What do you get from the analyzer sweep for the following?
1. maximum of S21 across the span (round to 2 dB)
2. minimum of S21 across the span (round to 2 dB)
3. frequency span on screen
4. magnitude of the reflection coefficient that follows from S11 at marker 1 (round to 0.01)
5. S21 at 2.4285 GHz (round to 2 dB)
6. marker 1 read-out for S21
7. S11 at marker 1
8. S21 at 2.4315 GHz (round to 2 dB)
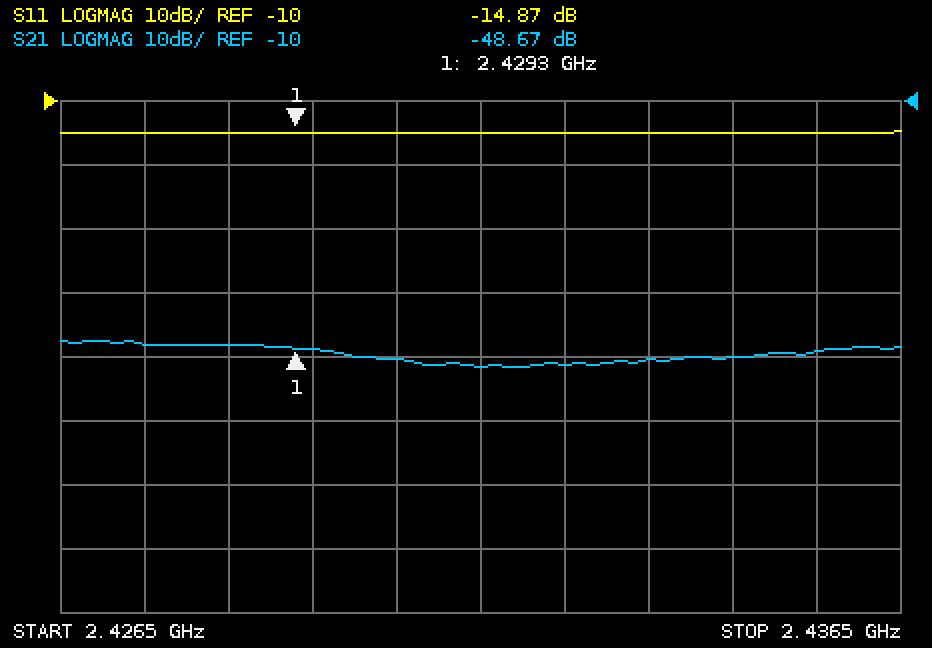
-48 dB
-52 dB
10 MHz
0.18
-48 dB
-48.67 dB
-14.87 dB
-52 dB
